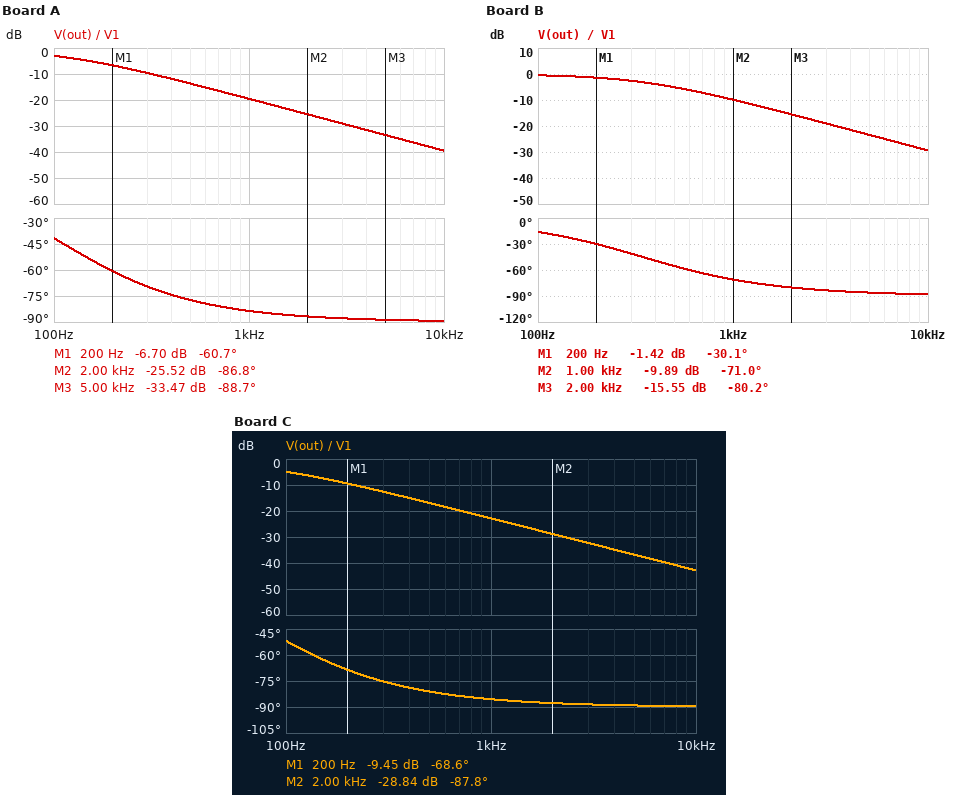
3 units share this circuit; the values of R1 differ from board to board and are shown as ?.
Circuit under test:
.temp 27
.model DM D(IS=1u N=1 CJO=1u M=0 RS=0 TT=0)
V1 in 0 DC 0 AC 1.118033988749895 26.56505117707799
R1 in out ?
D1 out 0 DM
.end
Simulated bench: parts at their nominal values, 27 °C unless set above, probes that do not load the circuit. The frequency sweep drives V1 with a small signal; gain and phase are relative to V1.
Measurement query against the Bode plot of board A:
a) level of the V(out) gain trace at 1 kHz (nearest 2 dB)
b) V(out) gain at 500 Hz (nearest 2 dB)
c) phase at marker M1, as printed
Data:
-20 dB
-14 dB
-60.7 deg
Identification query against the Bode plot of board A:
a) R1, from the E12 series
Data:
1.5 kΩ
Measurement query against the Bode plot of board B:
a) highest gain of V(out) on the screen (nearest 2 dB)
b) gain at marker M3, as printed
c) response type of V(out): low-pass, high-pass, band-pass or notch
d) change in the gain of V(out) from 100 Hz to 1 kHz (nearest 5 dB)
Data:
0 dB
-15.55 dB
low-pass
-10 dB
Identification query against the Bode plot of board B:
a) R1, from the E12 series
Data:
470 Ω
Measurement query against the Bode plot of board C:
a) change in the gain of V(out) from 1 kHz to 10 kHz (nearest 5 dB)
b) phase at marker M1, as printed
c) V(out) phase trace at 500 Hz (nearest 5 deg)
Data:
-20 dB
-68.6 deg
-80 deg
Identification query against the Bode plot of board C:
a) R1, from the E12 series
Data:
2.2 kΩ
